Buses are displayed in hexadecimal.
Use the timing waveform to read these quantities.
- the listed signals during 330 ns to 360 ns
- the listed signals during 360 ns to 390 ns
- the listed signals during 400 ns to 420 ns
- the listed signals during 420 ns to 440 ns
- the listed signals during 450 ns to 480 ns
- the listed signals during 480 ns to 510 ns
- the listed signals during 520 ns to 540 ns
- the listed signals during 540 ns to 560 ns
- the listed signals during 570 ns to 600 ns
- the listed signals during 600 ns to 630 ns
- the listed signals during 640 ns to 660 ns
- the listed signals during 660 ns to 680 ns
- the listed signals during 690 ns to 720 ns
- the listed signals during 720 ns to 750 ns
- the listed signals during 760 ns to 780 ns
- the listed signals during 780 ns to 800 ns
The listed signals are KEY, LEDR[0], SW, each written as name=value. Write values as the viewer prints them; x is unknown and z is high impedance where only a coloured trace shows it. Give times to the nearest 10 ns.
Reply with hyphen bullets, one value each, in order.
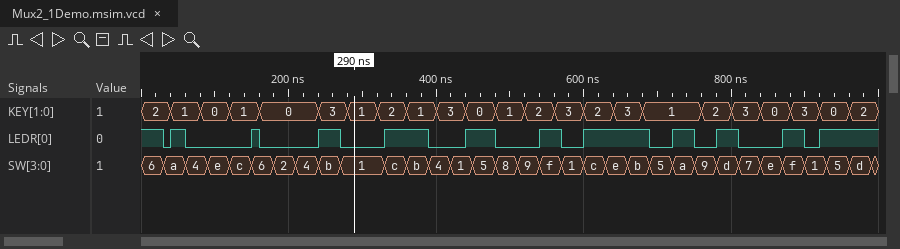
- KEY=2, LEDR[0]=1, SW=c
- KEY=1, LEDR[0]=1, SW=b
- KEY=3, LEDR[0]=0, SW=4
- KEY=3, LEDR[0]=0, SW=1
- KEY=0, LEDR[0]=1, SW=5
- KEY=1, LEDR[0]=0, SW=8
- KEY=2, LEDR[0]=0, SW=9
- KEY=2, LEDR[0]=1, SW=f
- KEY=3, LEDR[0]=0, SW=1
- KEY=2, LEDR[0]=1, SW=c
- KEY=3, LEDR[0]=1, SW=e
- KEY=3, LEDR[0]=1, SW=b
- KEY=1, LEDR[0]=0, SW=5
- KEY=1, LEDR[0]=1, SW=a
- KEY=2, LEDR[0]=0, SW=9
- KEY=2, LEDR[0]=1, SW=d
